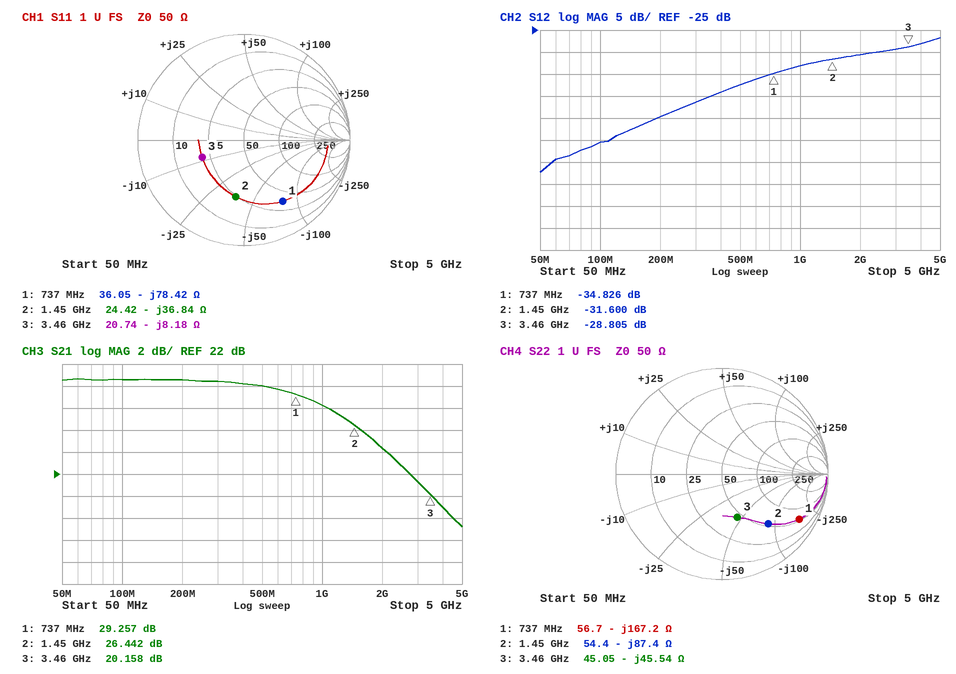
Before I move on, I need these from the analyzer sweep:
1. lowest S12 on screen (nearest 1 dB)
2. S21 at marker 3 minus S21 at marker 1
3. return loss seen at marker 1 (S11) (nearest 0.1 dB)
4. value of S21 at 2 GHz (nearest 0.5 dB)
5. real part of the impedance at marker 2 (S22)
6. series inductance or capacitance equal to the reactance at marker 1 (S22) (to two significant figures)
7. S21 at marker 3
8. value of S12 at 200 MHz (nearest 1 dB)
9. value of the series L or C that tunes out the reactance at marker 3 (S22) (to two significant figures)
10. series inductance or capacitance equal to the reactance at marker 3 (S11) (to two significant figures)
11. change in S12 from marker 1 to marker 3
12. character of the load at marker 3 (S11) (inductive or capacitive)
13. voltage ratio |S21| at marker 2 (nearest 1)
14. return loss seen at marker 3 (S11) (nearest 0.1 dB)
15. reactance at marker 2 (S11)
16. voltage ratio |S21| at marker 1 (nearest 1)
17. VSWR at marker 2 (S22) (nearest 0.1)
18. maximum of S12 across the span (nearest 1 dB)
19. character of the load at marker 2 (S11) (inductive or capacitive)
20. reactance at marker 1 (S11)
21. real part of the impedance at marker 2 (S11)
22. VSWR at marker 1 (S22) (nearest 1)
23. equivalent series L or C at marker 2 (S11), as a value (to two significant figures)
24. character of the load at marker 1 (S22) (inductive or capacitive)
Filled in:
-57 dB
-9.099 dB
3.3 dB
24.5 dB
54.4 Ω
1.3 pF
20.158 dB
-45 dB
2.1 nH
5.6 pF
6.021 dB
capacitive
21
7.4 dB
-36.84 Ω
29
4.6
-27 dB
capacitive
-78.42 Ω
24.42 Ω
12
3.0 pF
capacitive
